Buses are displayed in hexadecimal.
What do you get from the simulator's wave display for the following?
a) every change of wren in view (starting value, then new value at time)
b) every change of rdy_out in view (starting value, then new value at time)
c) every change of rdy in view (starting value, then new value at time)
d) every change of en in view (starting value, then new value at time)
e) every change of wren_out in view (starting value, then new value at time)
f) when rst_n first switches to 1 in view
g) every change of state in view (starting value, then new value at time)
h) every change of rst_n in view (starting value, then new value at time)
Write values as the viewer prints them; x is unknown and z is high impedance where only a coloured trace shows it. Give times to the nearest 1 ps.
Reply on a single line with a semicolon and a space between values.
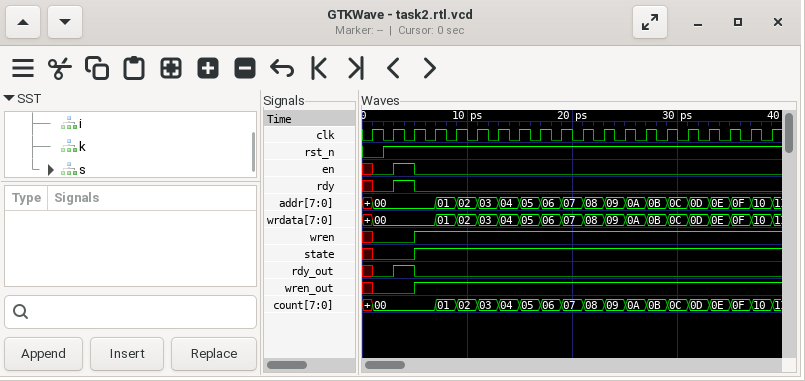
x, 0 at 1 ps, 1 at 5 ps; x, 0 at 1 ps, 1 at 3 ps, 0 at 5 ps; x, 0 at 1 ps, 1 at 3 ps, 0 at 5 ps; x, 0 at 1 ps, 1 at 3 ps, 0 at 5 ps; x, 0 at 1 ps, 1 at 5 ps; 2 ps; x, 0 at 1 ps, 1 at 5 ps; 0, 1 at 2 ps
